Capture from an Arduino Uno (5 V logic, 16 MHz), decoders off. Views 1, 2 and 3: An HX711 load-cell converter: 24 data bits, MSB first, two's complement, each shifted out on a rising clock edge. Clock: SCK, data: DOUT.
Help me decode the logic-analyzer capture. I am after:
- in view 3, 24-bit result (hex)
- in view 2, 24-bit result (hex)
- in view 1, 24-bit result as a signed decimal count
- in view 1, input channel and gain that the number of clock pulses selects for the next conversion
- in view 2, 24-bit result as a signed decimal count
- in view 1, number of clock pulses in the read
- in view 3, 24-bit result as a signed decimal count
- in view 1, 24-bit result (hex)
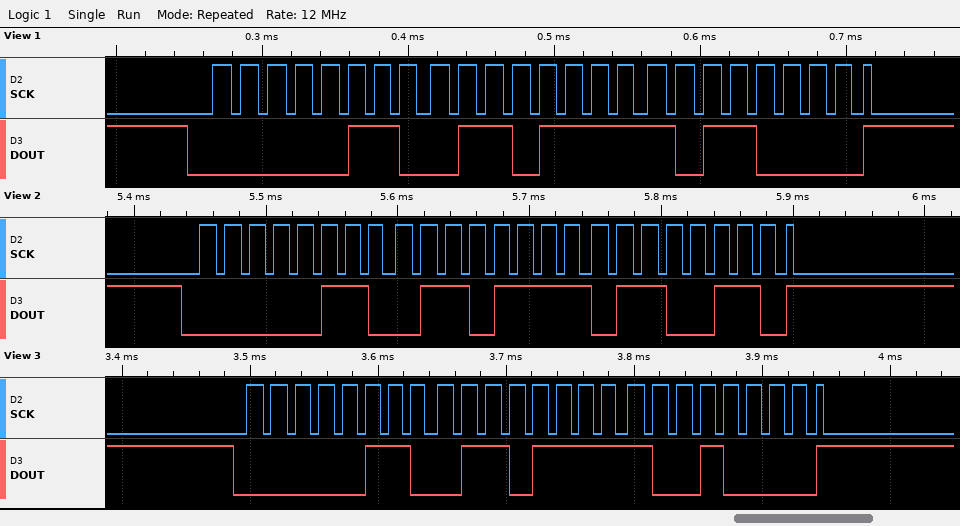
0x066F90
0x066F66
421808
channel A, gain 128
421734
25
421776
0x066FB0
